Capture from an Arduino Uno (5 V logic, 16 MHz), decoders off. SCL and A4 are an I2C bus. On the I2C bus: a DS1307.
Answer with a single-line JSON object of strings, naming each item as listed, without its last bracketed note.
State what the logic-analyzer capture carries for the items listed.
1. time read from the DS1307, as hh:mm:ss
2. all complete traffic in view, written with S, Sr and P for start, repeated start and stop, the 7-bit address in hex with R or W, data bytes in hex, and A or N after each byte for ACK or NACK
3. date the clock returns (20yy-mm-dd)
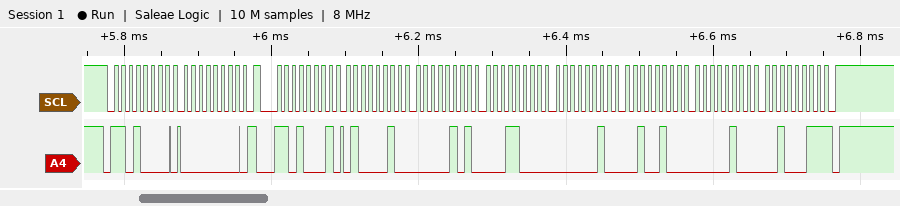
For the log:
{"time read from the DS1307, as hh:mm:ss": "18:05:42", "all complete traffic in view, written with S, Sr and P for start, repeated start and stop, the 7-bit address in hex with R or W, data bytes in hex, and A or N after each byte for ACK or NACK": "S 68W A 00 A Sr 68R A 42 A 05 A 18 A 02 A 24 A 04 A 23 N P", "date the clock returns": "2023-04-24"}
